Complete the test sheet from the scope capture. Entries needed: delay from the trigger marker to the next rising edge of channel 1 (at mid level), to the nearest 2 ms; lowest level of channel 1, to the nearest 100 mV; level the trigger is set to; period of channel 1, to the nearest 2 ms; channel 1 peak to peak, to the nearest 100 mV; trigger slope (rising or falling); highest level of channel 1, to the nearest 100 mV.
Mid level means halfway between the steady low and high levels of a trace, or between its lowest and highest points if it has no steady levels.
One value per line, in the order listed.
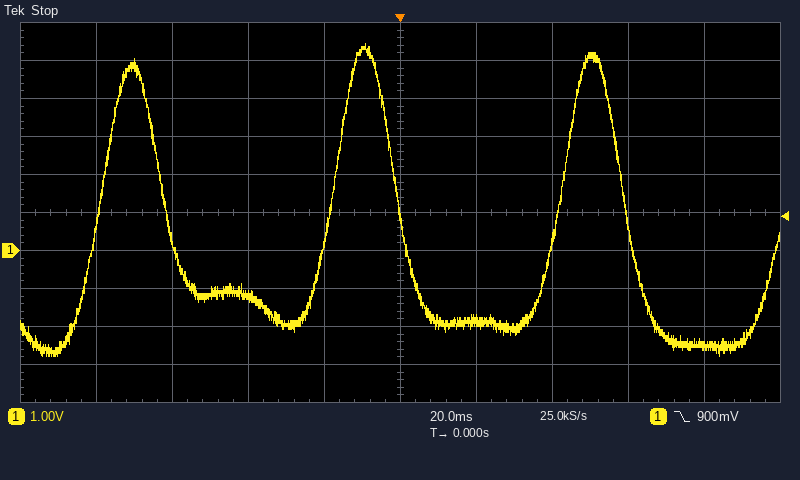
42 ms
-2.8 V
900 mV
60 ms
8.2 V
falling
5.4 V
